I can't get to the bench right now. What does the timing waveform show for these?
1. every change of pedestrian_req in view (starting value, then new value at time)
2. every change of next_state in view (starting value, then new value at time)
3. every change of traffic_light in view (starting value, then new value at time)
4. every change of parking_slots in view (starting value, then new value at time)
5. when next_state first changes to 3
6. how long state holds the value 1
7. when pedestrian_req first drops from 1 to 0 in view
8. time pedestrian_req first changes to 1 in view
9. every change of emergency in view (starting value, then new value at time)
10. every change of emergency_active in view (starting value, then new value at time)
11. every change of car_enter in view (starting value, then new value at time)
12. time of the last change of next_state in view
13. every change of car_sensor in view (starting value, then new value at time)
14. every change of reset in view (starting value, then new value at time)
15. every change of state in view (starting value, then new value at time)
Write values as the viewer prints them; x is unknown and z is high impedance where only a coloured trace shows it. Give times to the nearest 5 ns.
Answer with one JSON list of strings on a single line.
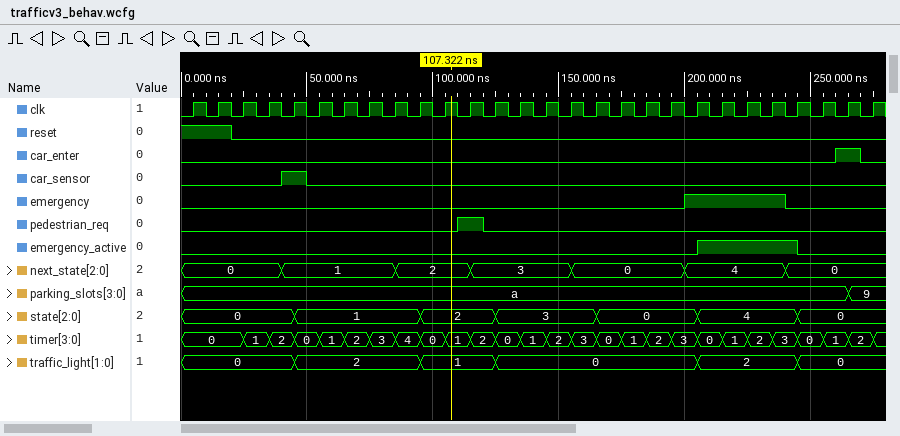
["0, 1 at 110 ns, 0 at 120 ns", "0, 1 at 40 ns, 2 at 85 ns, 3 at 115 ns, 0 at 155 ns, 4 at 200 ns, 0 at 240 ns", "0, 2 at 45 ns, 1 at 95 ns, 0 at 125 ns, 2 at 205 ns, 0 at 245 ns", "a, 9 at 265 ns", "115 ns", "50 ns", "120 ns", "110 ns", "0, 1 at 200 ns, 0 at 240 ns", "0, 1 at 205 ns, 0 at 245 ns", "0, 1 at 260 ns, 0 at 270 ns", "240 ns", "0, 1 at 40 ns, 0 at 50 ns", "1, 0 at 20 ns", "0, 1 at 45 ns, 2 at 95 ns, 3 at 125 ns, 0 at 165 ns, 4 at 205 ns, 0 at 245 ns"]
